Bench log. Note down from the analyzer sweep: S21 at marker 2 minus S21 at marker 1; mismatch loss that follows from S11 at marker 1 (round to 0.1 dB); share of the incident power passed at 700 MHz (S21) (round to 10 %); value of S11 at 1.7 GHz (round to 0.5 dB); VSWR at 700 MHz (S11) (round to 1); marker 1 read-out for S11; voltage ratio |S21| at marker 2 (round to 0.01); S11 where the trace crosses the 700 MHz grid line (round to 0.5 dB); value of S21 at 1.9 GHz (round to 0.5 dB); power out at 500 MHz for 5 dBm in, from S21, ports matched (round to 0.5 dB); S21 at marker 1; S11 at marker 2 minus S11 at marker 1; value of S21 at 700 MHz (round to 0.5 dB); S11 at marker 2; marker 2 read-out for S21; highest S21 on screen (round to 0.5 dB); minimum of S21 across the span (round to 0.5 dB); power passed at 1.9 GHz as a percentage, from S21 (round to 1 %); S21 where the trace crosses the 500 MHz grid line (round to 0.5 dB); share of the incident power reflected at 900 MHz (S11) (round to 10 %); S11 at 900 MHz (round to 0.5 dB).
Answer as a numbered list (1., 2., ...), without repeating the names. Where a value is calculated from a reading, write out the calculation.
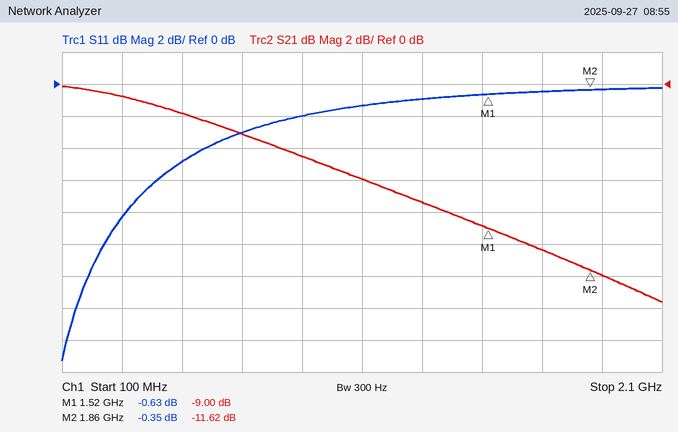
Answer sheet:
1. -11.62 − (-9) = -2.62 dB
2. −10 log10(1 − 10^(-0.63/10)) ≈ 8.7 dB
3. 10^(-3/10) ≈ 50 %
4. -0.5 dB
5. |Γ| = 10^(-3/20) = 0.7079; VSWR = (1 + 0.7079)/(1 − 0.7079) ≈ 6
6. -0.63 dB
7. 10^(-11.62/20) ≈ 0.26
8. -3.0 dB
9. -12.0 dB
10. 5 dBm + (-2.0 dB) = 3.0 dBm
11. -9.00 dB
12. -0.35 − (-0.63) = 0.28 dB
13. -3.0 dB
14. -0.35 dB
15. -11.62 dB
16. 0.0 dB
17. -13.5 dB
18. 10^(-12/10) ≈ 6 %
19. -2.0 dB
20. 10^(-2/10) ≈ 63.1 %, so 60 % to the nearest 10 %
21. -2.0 dB
